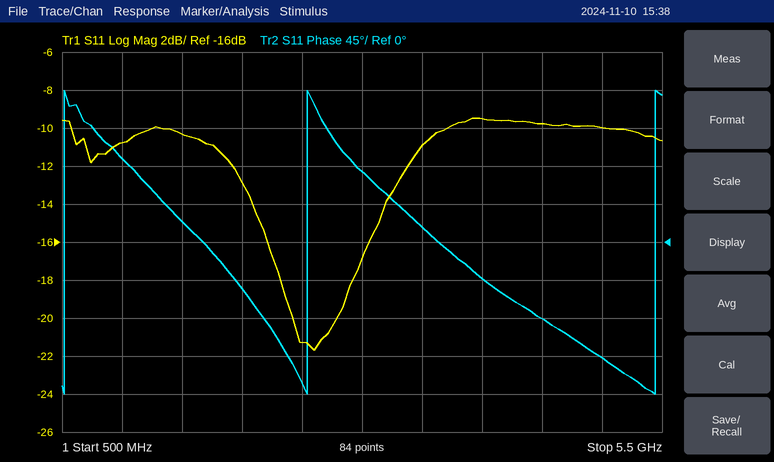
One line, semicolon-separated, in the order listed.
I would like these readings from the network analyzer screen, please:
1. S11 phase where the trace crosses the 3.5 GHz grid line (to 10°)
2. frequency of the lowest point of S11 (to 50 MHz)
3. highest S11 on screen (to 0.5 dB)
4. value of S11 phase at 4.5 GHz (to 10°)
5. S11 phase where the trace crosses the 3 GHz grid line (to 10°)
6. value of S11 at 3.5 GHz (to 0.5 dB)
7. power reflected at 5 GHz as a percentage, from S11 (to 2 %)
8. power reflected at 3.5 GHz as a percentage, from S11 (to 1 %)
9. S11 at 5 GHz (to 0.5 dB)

20°; 2.60 GHz; -9.5 dB; -90°; 80°; -11.0 dB; 10 %; 8 %; -10.0 dB
